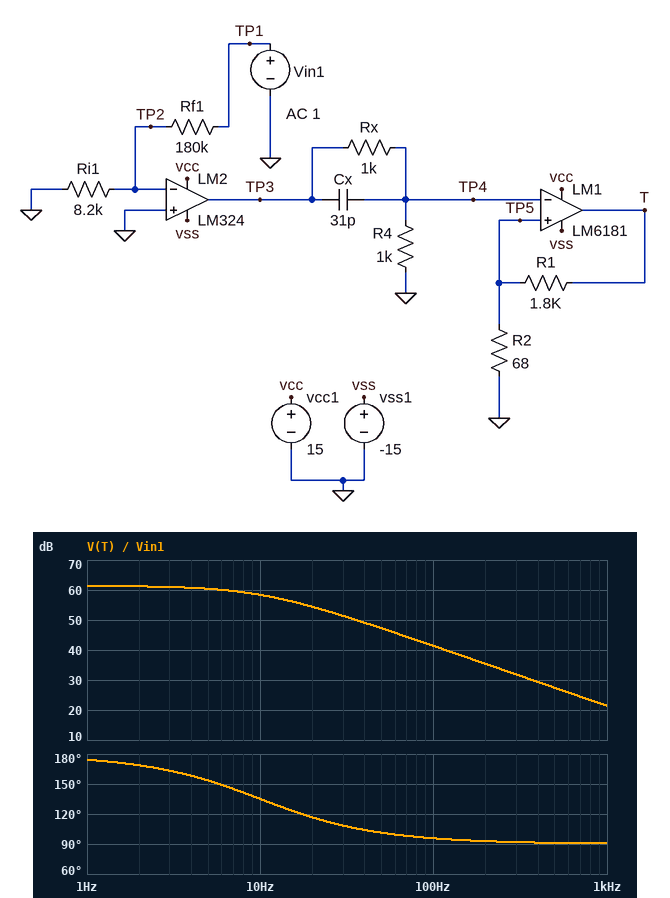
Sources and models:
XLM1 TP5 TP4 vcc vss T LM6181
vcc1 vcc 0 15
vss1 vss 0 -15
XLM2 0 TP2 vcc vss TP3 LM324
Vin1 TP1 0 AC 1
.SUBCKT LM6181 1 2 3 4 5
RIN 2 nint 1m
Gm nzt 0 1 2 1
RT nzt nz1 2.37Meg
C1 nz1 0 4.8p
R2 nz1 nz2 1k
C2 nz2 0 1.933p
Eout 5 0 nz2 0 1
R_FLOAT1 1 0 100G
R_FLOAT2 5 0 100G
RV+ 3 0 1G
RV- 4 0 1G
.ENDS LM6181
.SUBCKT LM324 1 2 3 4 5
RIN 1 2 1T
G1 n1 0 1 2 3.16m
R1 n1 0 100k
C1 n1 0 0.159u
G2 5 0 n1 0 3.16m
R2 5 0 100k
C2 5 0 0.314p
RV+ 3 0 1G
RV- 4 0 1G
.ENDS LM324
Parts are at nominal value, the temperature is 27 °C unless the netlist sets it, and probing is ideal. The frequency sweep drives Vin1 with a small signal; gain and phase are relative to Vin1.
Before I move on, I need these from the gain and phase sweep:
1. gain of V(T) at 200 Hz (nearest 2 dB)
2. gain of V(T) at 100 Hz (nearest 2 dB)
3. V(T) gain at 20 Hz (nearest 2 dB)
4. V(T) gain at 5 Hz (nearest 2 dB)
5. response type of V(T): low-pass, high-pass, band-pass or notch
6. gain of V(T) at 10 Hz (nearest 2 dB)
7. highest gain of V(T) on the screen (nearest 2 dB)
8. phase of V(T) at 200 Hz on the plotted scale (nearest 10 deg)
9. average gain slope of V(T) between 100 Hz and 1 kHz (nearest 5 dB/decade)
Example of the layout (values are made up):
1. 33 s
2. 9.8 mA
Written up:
1. 36 dB
2. 42 dB
3. 54 dB
4. 60 dB
5. low-pass
6. 58 dB
7. 62 dB
8. 90 deg
9. -20 dB/decade
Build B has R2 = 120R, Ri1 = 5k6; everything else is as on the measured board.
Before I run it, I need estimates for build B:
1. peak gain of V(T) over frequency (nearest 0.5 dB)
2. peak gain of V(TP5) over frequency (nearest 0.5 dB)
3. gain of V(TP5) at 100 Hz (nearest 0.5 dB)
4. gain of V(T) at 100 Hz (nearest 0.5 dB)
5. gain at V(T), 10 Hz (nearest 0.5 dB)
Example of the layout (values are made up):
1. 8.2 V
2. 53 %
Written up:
1. 53.5 dB
2. 29.5 dB
3. 9.5 dB
4. 33.5 dB
5. 50.5 dB
